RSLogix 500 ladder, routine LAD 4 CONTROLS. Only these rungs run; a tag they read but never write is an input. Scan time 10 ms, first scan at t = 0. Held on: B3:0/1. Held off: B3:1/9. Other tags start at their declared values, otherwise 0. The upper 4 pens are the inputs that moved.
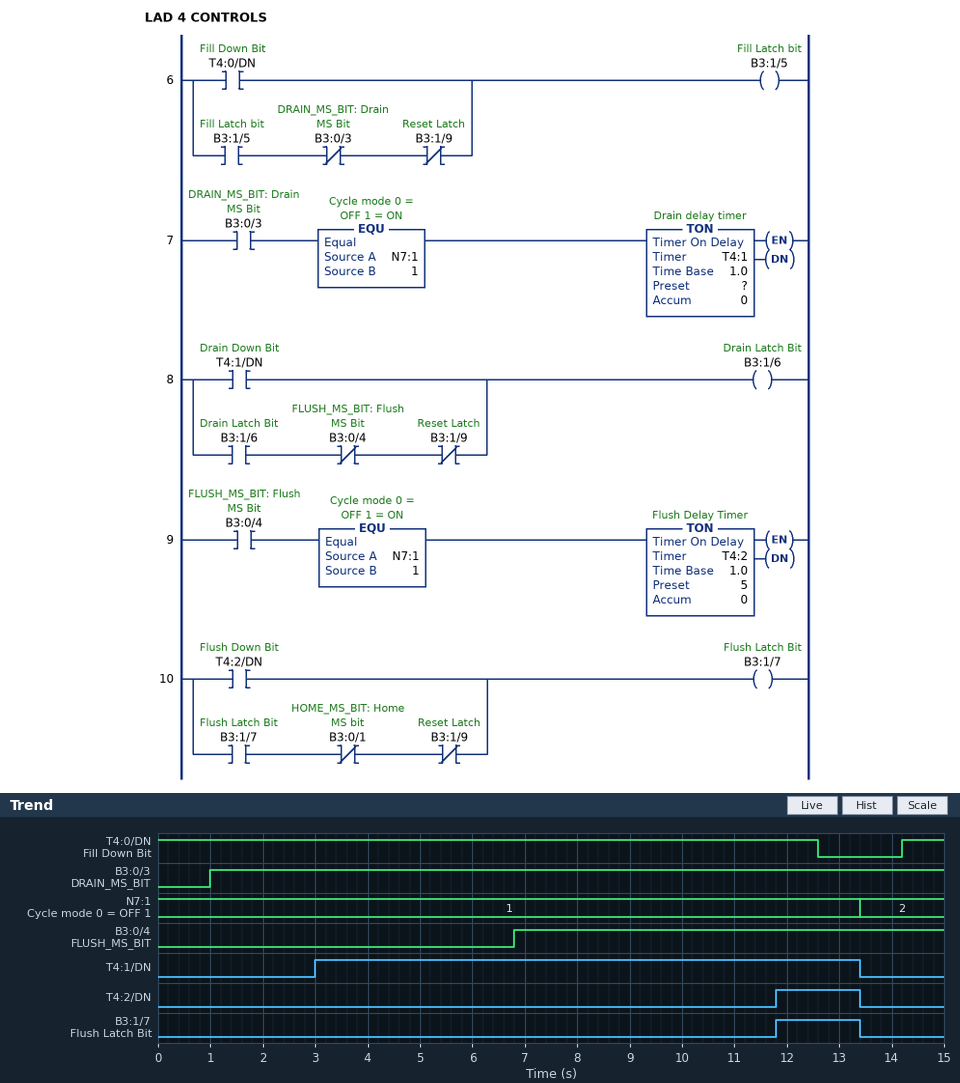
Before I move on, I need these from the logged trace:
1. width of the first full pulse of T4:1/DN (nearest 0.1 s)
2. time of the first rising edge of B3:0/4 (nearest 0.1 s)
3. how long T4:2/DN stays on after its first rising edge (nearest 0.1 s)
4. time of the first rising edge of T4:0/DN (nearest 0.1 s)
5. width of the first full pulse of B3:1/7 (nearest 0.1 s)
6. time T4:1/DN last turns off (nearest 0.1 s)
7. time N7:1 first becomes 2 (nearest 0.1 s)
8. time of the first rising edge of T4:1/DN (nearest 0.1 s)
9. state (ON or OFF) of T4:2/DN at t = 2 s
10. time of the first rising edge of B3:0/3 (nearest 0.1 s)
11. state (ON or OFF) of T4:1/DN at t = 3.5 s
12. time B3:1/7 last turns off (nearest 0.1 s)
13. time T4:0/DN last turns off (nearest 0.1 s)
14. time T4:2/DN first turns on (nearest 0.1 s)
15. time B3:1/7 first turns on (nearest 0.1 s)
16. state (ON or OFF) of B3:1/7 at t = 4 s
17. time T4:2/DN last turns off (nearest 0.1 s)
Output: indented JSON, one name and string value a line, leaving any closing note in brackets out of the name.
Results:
{
  "width of the first full pulse of T4:1/DN": "10.4 s",
  "time of the first rising edge of B3:0/4": "6.8 s",
  "how long T4:2/DN stays on after its first rising edge": "1.6 s",
  "time of the first rising edge of T4:0/DN": "14.2 s",
  "width of the first full pulse of B3:1/7": "1.6 s",
  "time T4:1/DN last turns off": "13.4 s",
  "time N7:1 first becomes 2": "13.4 s",
  "time of the first rising edge of T4:1/DN": "3.0 s",
  "state (ON or OFF) of T4:2/DN at t = 2 s": "OFF",
  "time of the first rising edge of B3:0/3": "1.0 s",
  "state (ON or OFF) of T4:1/DN at t = 3.5 s": "ON",
  "time B3:1/7 last turns off": "13.4 s",
  "time T4:0/DN last turns off": "12.6 s",
  "time T4:2/DN first turns on": "11.8 s",
  "time B3:1/7 first turns on": "11.8 s",
  "state (ON or OFF) of B3:1/7 at t = 4 s": "OFF",
  "time T4:2/DN last turns off": "13.4 s"
}
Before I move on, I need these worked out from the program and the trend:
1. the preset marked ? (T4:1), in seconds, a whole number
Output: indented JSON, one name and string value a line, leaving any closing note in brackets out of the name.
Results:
{
  "the preset marked ? (T4:1), in seconds, a whole number": "2 s"
}
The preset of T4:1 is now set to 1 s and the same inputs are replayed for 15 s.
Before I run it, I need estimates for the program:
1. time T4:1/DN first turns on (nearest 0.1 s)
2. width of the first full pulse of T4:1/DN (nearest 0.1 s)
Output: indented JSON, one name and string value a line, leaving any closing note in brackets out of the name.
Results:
{
  "time T4:1/DN first turns on": "2.0 s",
  "width of the first full pulse of T4:1/DN": "11.4 s"
}
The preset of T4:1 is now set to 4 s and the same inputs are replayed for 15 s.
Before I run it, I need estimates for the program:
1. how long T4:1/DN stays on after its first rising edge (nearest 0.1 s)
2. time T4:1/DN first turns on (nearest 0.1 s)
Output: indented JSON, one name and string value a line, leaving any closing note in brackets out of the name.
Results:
{
  "how long T4:1/DN stays on after its first rising edge": "8.4 s",
  "time T4:1/DN first turns on": "5.0 s"
}
